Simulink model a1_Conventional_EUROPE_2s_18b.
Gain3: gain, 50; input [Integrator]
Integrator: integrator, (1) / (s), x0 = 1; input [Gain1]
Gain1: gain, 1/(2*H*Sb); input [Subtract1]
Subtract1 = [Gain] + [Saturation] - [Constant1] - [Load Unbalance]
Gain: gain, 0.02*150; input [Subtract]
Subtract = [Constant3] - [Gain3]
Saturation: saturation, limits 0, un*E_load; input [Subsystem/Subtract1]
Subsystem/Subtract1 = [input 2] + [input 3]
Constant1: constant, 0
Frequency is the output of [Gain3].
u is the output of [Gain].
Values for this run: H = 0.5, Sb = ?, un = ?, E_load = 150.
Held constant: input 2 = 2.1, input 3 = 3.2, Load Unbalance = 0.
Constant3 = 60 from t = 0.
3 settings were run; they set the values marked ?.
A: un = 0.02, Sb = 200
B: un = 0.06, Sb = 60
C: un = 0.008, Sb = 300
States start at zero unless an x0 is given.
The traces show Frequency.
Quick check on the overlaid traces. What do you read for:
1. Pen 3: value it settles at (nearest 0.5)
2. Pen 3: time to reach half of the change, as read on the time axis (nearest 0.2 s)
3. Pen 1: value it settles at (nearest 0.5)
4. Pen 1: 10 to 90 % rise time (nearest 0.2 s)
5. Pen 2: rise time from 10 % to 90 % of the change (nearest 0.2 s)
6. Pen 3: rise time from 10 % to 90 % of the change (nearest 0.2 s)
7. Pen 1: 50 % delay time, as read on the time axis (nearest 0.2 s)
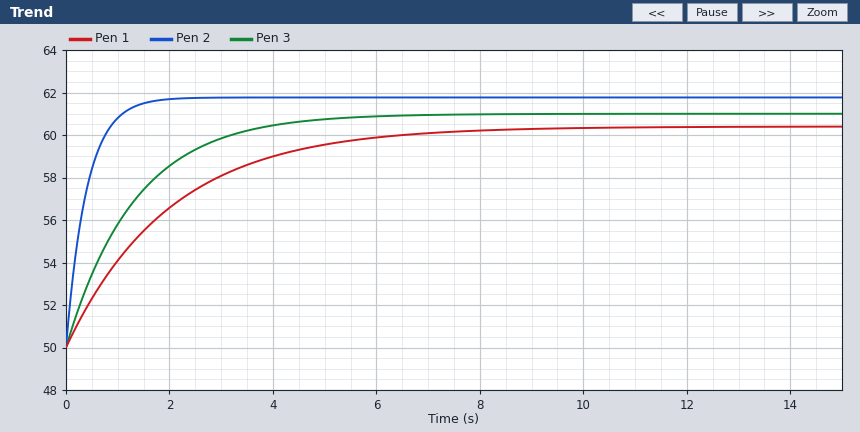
61.0
1.0 s
60.5
4.4 s
0.8 s
3.0 s
1.4 s
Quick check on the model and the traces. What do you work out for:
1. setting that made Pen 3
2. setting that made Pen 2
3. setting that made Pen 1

A
B
C
